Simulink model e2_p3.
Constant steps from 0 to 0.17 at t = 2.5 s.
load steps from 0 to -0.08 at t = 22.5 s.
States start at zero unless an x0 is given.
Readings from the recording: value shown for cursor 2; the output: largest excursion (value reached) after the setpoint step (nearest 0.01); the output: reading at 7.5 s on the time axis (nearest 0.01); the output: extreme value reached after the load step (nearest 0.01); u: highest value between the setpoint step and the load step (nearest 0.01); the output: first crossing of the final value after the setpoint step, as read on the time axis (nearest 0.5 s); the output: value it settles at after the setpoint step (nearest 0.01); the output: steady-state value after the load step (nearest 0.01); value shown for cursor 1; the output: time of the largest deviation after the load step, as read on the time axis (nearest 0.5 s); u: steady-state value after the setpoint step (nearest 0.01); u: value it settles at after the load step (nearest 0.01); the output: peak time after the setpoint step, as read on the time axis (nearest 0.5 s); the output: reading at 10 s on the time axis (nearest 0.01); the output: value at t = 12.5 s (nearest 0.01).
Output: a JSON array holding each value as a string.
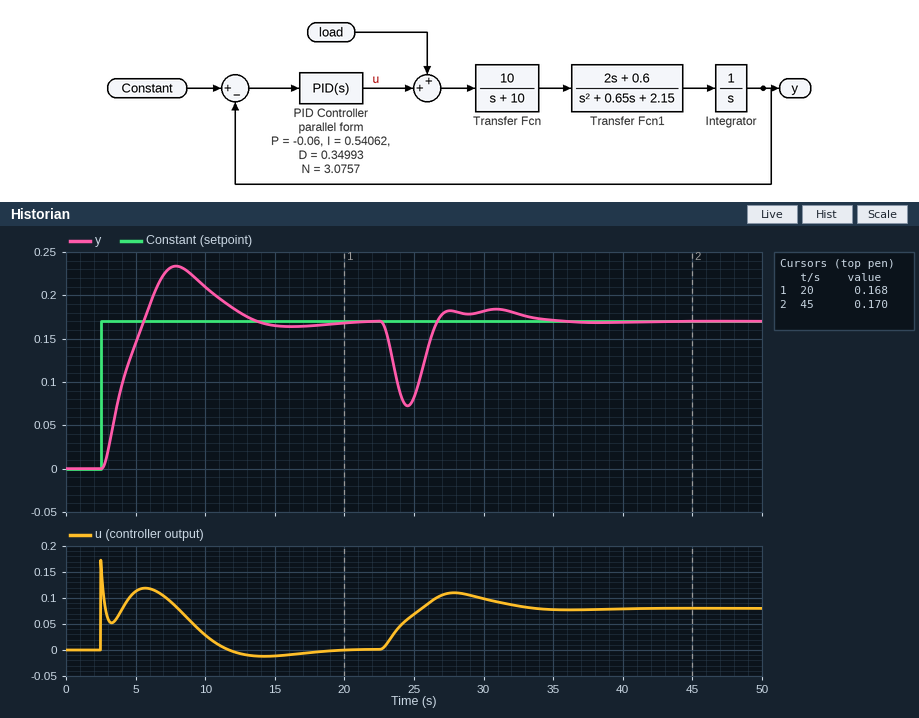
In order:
["0.170", "0.23", "0.23", "0.07", "0.17", "5.5 s", "0.17", "0.17", "0.168", "24.5 s", "0.00", "0.08", "8.0 s", "0.21", "0.18"]
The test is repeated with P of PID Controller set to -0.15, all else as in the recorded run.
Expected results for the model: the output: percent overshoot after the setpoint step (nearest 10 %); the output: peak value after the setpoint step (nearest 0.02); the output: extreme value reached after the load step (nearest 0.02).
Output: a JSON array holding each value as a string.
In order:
["50 %", "0.24", "0.06"]
